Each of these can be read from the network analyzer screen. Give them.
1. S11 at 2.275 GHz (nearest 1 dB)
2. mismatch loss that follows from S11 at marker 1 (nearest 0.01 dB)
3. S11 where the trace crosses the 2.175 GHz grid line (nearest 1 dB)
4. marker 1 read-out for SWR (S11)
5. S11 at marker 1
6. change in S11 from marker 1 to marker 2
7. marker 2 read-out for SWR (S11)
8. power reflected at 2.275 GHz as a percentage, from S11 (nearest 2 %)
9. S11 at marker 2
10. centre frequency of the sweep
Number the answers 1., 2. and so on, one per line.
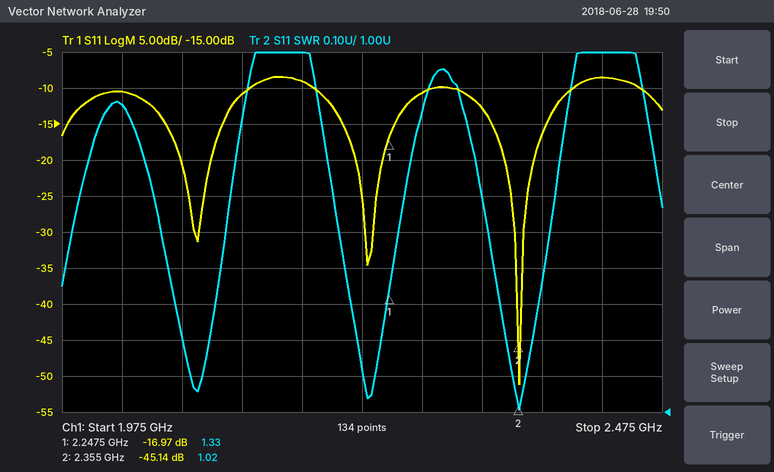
1. -11 dB
2. 0.09 dB
3. -9 dB
4. 1.33
5. -16.97 dB
6. -28.17 dB
7. 1.02
8. 8 %
9. -45.14 dB
10. 2.225 GHz
